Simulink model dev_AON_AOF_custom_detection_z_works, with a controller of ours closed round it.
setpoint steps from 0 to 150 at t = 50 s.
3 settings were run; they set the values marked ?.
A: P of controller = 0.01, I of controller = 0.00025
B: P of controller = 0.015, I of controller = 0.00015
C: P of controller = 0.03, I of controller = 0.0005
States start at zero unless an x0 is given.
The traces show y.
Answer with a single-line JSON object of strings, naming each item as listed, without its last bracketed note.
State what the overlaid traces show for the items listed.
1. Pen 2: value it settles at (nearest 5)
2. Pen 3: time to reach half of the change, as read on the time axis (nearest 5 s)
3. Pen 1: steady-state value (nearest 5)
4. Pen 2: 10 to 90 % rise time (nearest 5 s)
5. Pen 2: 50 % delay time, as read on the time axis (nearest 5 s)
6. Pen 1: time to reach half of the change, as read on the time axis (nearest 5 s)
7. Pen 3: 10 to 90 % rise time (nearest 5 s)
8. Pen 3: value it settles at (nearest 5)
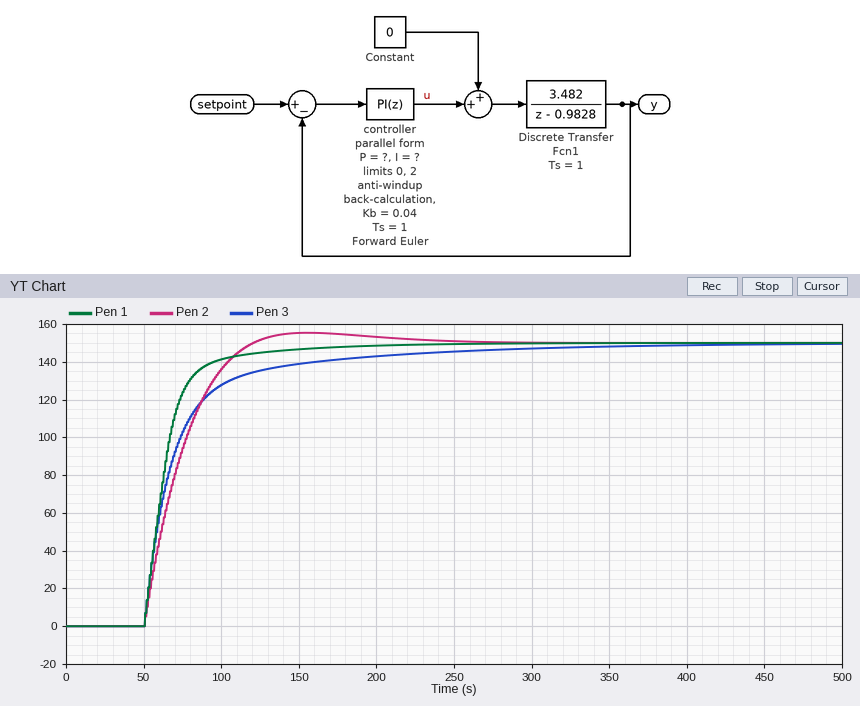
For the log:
{"Pen 2: value it settles at": "150", "Pen 3: time to reach half of the change, as read on the time axis": "65 s", "Pen 1: steady-state value": "150", "Pen 2: 10 to 90 % rise time": "45 s", "Pen 2: 50 % delay time, as read on the time axis": "70 s", "Pen 1: time to reach half of the change, as read on the time axis": "60 s", "Pen 3: 10 to 90 % rise time": "70 s", "Pen 3: value it settles at": "150"}
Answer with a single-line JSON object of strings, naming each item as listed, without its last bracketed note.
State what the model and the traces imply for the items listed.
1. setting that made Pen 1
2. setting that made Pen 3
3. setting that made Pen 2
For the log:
{"setting that made Pen 1": "C", "setting that made Pen 3": "B", "setting that made Pen 2": "A"}
